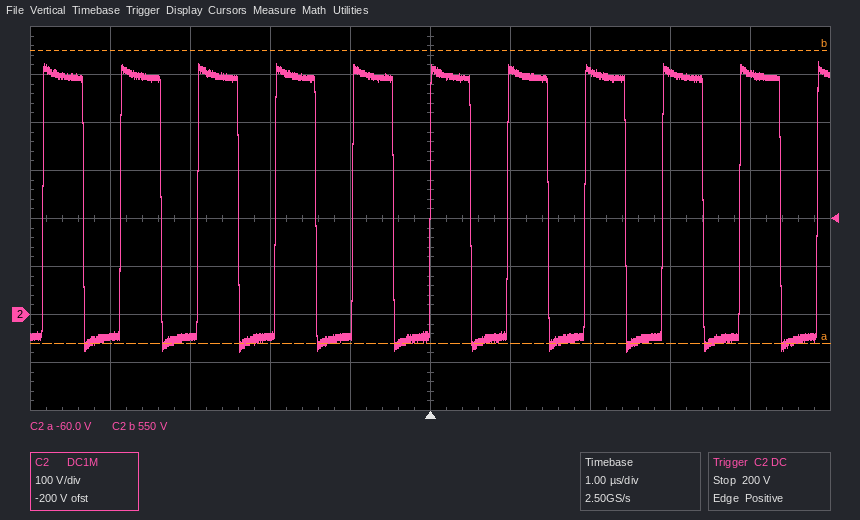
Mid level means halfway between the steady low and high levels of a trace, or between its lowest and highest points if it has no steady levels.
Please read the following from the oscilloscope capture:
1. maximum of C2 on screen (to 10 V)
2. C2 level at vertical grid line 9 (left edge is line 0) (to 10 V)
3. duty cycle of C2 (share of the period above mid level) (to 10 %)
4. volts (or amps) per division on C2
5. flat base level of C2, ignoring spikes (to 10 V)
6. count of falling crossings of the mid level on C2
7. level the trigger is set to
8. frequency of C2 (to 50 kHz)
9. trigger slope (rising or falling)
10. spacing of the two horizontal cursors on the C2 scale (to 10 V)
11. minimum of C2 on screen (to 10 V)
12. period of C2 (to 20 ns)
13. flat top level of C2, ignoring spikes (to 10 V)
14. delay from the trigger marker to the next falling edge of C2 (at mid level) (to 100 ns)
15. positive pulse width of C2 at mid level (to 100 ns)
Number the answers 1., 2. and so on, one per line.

1. 530 V
2. 500 V
3. 50 %
4. 100 V
5. -50 V
6. 10
7. 200 V
8. 1.05 MHz
9. rising
10. 610 V
11. -80 V
12. 960 ns
13. 490 V
14. 500 ns
15. 500 ns
